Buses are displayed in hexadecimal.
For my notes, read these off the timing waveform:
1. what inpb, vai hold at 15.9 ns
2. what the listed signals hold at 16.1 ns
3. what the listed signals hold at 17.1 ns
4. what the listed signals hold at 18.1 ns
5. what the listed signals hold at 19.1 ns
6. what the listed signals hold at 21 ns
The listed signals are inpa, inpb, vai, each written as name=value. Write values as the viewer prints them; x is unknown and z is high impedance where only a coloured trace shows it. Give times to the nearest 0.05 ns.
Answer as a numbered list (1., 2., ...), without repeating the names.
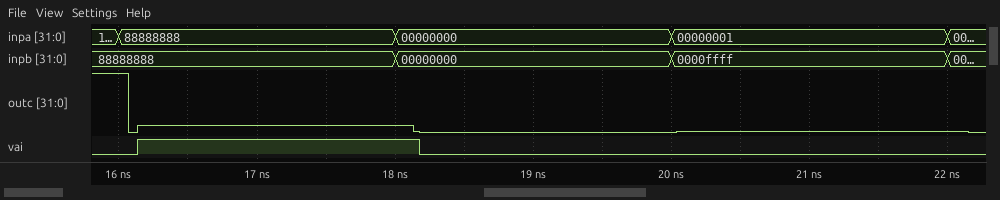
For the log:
1. inpb=88888888, vai=0
2. inpa=88888888, inpb=88888888, vai=0
3. inpa=88888888, inpb=88888888, vai=1
4. inpa=00000000, inpb=00000000, vai=1
5. inpa=00000000, inpb=00000000, vai=0
6. inpa=00000001, inpb=0000ffff, vai=0
